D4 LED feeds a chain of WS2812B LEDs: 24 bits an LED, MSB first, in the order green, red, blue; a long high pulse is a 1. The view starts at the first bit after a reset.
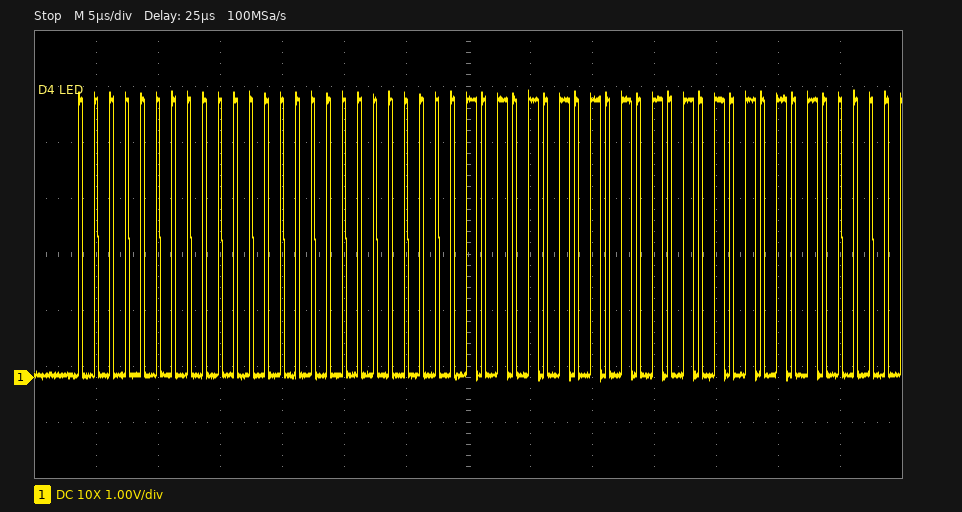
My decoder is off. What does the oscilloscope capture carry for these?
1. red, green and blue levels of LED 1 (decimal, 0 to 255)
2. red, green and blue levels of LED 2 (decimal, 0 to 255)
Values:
0, 0, 0
85, 85, 85
